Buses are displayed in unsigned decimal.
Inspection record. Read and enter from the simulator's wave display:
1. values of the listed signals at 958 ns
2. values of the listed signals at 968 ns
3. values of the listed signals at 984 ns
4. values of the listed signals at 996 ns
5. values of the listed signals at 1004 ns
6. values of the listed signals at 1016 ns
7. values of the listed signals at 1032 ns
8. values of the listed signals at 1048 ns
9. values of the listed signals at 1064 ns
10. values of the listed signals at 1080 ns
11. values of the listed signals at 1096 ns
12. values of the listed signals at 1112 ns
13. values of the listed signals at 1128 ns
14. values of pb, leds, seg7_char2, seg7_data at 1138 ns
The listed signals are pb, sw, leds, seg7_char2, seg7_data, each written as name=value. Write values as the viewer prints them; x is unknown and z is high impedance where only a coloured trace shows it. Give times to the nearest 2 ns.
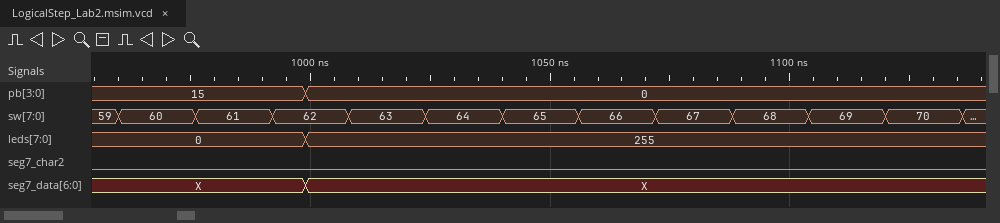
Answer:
pb=15, sw=59, leds=0, seg7_char2=0, seg7_data=X
pb=15, sw=60, leds=0, seg7_char2=0, seg7_data=X
pb=15, sw=61, leds=0, seg7_char2=0, seg7_data=X
pb=15, sw=62, leds=0, seg7_char2=0, seg7_data=X
pb=0, sw=62, leds=255, seg7_char2=0, seg7_data=X
pb=0, sw=63, leds=255, seg7_char2=0, seg7_data=X
pb=0, sw=64, leds=255, seg7_char2=0, seg7_data=X
pb=0, sw=65, leds=255, seg7_char2=0, seg7_data=X
pb=0, sw=66, leds=255, seg7_char2=0, seg7_data=X
pb=0, sw=67, leds=255, seg7_char2=0, seg7_data=X
pb=0, sw=68, leds=255, seg7_char2=0, seg7_data=X
pb=0, sw=69, leds=255, seg7_char2=0, seg7_data=X
pb=0, sw=70, leds=255, seg7_char2=0, seg7_data=X
pb=0, leds=255, seg7_char2=0, seg7_data=X
